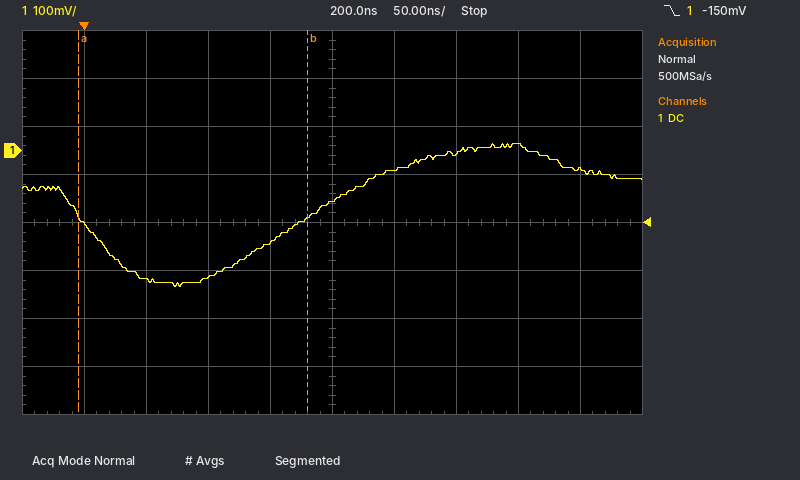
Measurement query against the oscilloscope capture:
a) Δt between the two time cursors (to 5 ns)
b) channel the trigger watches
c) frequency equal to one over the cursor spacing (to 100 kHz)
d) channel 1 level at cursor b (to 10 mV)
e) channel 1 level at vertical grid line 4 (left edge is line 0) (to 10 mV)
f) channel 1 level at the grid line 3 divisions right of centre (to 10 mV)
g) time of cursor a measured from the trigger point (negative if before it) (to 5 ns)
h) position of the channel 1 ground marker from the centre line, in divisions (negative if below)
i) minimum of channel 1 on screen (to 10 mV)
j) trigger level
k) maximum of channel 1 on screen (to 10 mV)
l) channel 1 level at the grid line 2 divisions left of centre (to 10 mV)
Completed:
185 ns
channel 1
5.4 MHz
-140 mV
-190 mV
10 mV
-5 ns
+1.5 div
-280 mV
-150 mV
10 mV
-260 mV
